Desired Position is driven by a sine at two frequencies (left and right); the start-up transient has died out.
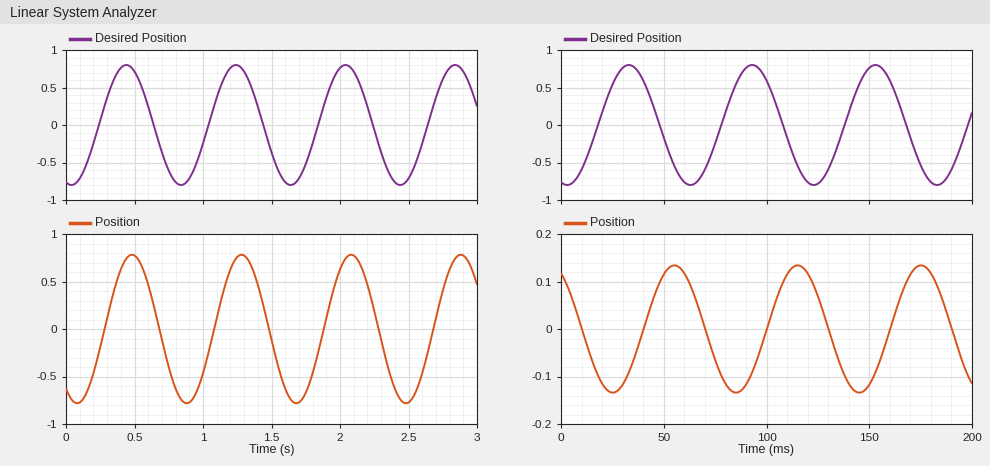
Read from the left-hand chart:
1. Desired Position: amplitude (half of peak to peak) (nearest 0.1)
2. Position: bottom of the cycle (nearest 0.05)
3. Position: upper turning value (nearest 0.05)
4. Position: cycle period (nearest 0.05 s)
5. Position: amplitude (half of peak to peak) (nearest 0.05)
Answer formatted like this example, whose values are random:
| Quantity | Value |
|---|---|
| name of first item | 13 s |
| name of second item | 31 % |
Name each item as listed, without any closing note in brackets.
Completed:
| Quantity | Value |
|---|---|
| Desired Position: amplitude (half of peak to peak) | 0.8 |
| Position: bottom of the cycle | -0.80 |
| Position: upper turning value | 0.80 |
| Position: cycle period | 0.80 s |
| Position: amplitude (half of peak to peak) | 0.80 |
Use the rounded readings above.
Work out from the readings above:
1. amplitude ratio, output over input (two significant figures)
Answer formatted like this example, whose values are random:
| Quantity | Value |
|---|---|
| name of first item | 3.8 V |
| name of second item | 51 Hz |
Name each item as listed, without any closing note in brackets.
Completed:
| Quantity | Value |
|---|---|
| amplitude ratio, output over input | 1.0 |
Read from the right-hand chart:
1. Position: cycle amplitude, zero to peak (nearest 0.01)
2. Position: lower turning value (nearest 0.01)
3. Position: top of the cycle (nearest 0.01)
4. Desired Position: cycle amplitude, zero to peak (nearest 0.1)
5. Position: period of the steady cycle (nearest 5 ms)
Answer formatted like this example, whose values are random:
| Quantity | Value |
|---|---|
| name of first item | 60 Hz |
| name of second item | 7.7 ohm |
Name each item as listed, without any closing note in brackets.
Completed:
| Quantity | Value |
|---|---|
| Position: cycle amplitude, zero to peak | 0.13 |
| Position: lower turning value | -0.13 |
| Position: top of the cycle | 0.13 |
| Desired Position: cycle amplitude, zero to peak | 0.8 |
| Position: period of the steady cycle | 60 ms |
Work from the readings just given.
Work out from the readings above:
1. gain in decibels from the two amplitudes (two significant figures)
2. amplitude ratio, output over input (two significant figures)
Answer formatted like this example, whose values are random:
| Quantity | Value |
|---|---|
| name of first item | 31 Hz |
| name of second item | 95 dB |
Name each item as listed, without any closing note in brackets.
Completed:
| Quantity | Value |
|---|---|
| gain in decibels from the two amplitudes | -16 dB |
| amplitude ratio, output over input | 0.16 |
